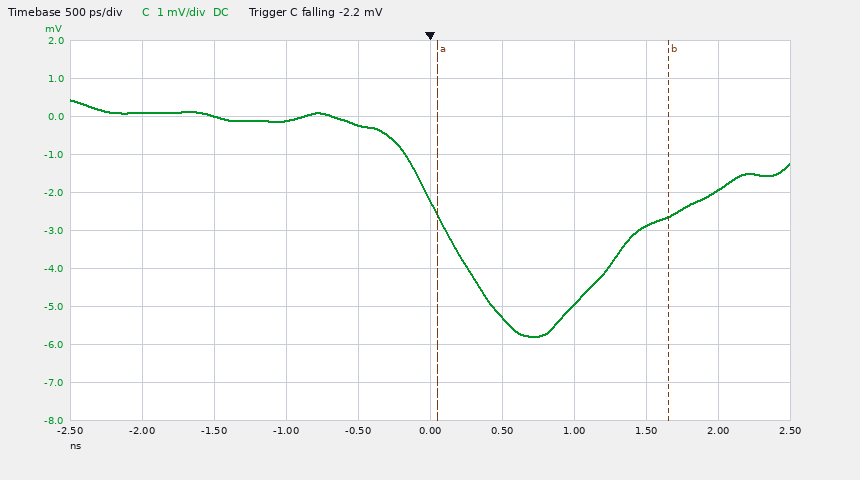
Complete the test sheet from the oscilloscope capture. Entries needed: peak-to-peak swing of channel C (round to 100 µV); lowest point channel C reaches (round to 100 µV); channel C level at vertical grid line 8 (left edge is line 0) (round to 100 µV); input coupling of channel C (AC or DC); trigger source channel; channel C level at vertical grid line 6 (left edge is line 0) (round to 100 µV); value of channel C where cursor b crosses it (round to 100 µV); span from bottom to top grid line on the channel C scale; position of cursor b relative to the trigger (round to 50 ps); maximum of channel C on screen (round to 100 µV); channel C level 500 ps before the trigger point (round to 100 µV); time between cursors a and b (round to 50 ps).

6.2 mV
-5.8 mV
-2.9 mV
DC
channel C
-5.3 mV
-2.6 mV
10 mV
+1.65 ns
400 µV
-200 µV
1.60 ns
